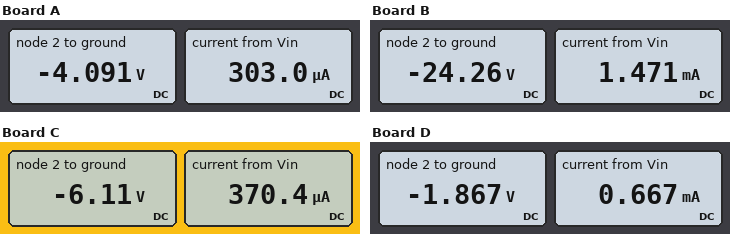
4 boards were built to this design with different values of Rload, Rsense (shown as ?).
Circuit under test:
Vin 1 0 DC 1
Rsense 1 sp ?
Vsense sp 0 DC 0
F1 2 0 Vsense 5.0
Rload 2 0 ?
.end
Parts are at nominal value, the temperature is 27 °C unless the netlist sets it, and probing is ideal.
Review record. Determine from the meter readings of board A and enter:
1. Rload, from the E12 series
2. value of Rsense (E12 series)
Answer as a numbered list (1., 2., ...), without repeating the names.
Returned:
1. 2.7 kΩ
2. 3.3 kΩ
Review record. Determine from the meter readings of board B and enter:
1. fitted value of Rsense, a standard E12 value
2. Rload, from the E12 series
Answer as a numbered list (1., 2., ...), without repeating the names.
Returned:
1. 680 Ω
2. 3.3 kΩ
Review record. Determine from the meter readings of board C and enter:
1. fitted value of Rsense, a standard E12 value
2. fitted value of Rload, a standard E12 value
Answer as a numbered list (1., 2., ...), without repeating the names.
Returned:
1. 2.7 kΩ
2. 3.3 kΩ
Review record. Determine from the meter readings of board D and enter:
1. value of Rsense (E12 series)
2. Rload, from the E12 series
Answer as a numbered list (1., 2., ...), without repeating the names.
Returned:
1. 1.5 kΩ
2. 560 Ω
